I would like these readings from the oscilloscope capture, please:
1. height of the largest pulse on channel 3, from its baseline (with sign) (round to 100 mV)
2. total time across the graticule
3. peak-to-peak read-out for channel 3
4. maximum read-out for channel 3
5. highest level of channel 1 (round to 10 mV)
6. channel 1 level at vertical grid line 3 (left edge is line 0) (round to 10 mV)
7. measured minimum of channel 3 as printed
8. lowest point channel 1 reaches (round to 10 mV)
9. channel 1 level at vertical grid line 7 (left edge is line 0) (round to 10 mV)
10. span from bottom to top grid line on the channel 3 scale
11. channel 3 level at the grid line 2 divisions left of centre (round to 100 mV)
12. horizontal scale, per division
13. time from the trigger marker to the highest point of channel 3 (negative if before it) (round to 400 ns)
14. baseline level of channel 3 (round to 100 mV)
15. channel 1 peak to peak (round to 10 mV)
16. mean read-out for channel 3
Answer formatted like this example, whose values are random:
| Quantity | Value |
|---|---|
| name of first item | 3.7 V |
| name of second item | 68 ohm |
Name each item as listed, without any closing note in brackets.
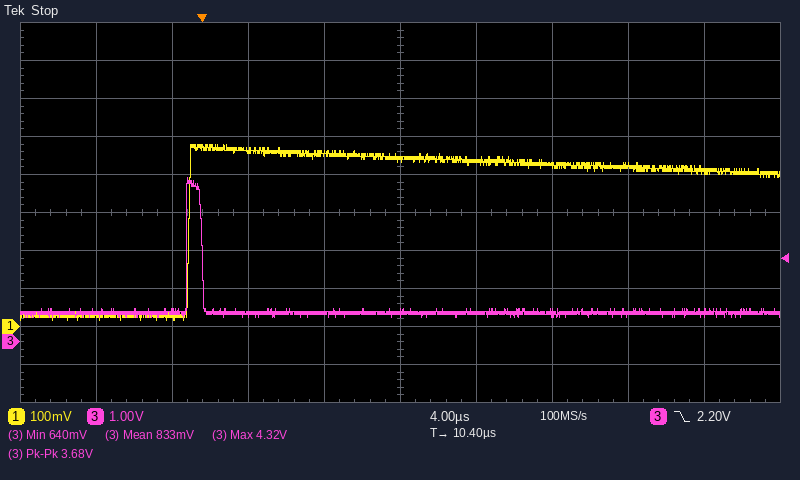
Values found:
| Quantity | Value |
|---|---|
| height of the largest pulse on channel 3, from its baseline (with sign) | +3.6 V |
| total time across the graticule | 40 µs |
| peak-to-peak read-out for channel 3 | 3.68 V |
| maximum read-out for channel 3 | 4.32 V |
| highest level of channel 1 | 480 mV |
| channel 1 level at vertical grid line 3 (left edge is line 0) | 460 mV |
| measured minimum of channel 3 as printed | 640 mV |
| lowest point channel 1 reaches | 20 mV |
| channel 1 level at vertical grid line 7 (left edge is line 0) | 420 mV |
| span from bottom to top grid line on the channel 3 scale | 10 V |
| channel 3 level at the grid line 2 divisions left of centre | 700 mV |
| horizontal scale, per division | 4 µs |
| time from the trigger marker to the highest point of channel 3 (negative if before it) | -800 ns |
| baseline level of channel 3 | 800 mV |
| channel 1 peak to peak | 460 mV |
| mean read-out for channel 3 | 833 mV |
